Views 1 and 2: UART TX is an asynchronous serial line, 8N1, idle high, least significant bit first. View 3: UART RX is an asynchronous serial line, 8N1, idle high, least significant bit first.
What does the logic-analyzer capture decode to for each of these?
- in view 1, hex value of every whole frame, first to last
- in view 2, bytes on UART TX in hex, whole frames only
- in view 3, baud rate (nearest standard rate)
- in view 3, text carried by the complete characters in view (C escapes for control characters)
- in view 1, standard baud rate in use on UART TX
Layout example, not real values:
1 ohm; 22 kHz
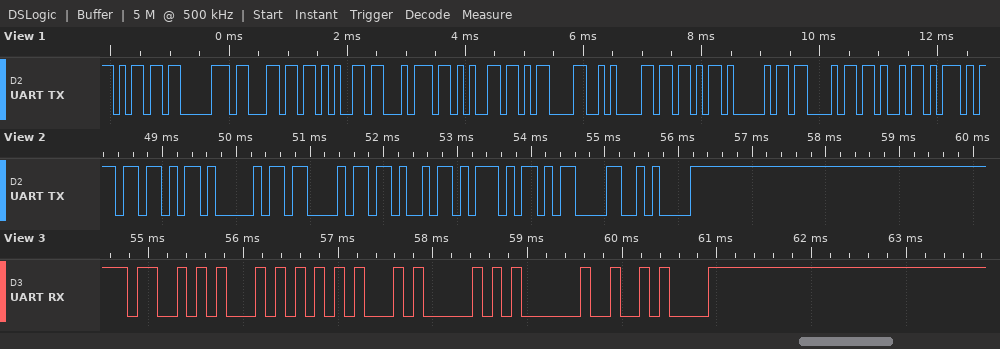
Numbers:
6D 70 6C 65 74 65 0D 0A 5B 41 43 4B 5D; 0x5B 0x41 0x43 0x4B 0x5D 0x0D 0x0A; 9600 baud; "STEP \n"; 9600 baud
